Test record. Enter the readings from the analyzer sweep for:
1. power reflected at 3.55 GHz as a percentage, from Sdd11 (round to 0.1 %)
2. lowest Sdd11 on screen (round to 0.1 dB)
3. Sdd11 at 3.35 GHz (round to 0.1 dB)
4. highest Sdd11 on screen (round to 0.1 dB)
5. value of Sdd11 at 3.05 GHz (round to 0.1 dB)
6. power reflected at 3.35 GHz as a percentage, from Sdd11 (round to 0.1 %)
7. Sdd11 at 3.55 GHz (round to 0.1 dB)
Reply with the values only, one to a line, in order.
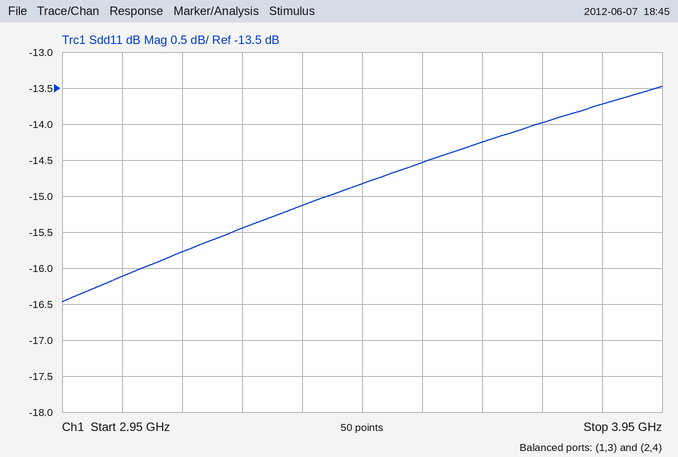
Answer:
3.5 %
-16.5 dB
-15.1 dB
-13.5 dB
-16.1 dB
3.1 %
-14.5 dB
